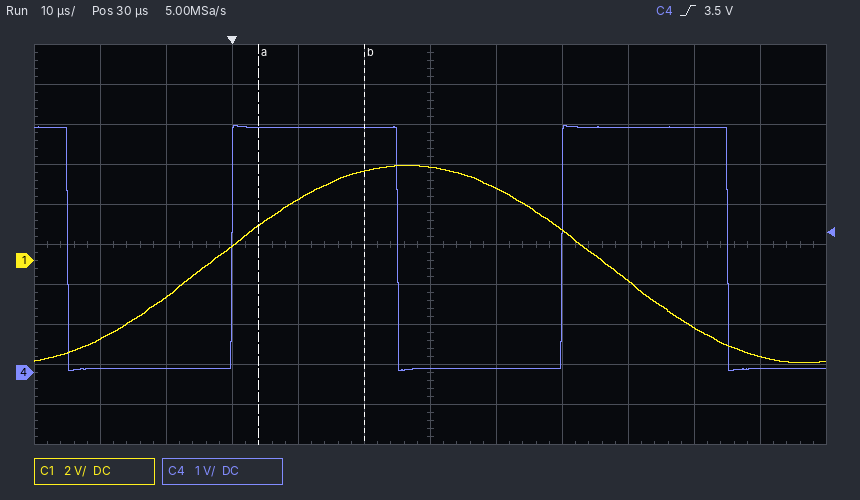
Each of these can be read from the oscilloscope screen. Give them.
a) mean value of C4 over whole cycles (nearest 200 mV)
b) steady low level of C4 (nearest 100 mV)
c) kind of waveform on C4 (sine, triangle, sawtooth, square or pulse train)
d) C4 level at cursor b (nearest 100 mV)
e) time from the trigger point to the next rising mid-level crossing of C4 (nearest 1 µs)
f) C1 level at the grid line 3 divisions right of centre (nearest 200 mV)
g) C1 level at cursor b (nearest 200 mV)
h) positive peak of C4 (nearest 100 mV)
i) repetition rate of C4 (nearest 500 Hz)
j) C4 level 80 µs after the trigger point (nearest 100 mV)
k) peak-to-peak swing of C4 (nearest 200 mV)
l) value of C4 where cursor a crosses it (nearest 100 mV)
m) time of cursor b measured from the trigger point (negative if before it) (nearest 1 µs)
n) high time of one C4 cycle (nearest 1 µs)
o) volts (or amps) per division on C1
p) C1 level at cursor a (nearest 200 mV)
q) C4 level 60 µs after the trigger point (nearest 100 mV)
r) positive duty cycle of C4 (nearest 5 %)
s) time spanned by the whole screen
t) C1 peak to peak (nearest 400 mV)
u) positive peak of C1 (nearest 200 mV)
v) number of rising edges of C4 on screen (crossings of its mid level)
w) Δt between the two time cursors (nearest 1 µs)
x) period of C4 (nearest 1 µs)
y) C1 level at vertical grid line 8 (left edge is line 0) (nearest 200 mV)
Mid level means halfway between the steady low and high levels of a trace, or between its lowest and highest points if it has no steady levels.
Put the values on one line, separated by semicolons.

3.2 V; 100 mV; square; 6.1 V; 50 µs; -1.0 V; 4.4 V; 6.2 V; 20.0 kHz; 100 mV; 6.2 V; 6.1 V; +20 µs; 25 µs; 2 V; 1.8 V; 6.1 V; 50 %; 120 µs; 10.0 V; 4.8 V; 2; 16 µs; 50 µs; 1.6 V
